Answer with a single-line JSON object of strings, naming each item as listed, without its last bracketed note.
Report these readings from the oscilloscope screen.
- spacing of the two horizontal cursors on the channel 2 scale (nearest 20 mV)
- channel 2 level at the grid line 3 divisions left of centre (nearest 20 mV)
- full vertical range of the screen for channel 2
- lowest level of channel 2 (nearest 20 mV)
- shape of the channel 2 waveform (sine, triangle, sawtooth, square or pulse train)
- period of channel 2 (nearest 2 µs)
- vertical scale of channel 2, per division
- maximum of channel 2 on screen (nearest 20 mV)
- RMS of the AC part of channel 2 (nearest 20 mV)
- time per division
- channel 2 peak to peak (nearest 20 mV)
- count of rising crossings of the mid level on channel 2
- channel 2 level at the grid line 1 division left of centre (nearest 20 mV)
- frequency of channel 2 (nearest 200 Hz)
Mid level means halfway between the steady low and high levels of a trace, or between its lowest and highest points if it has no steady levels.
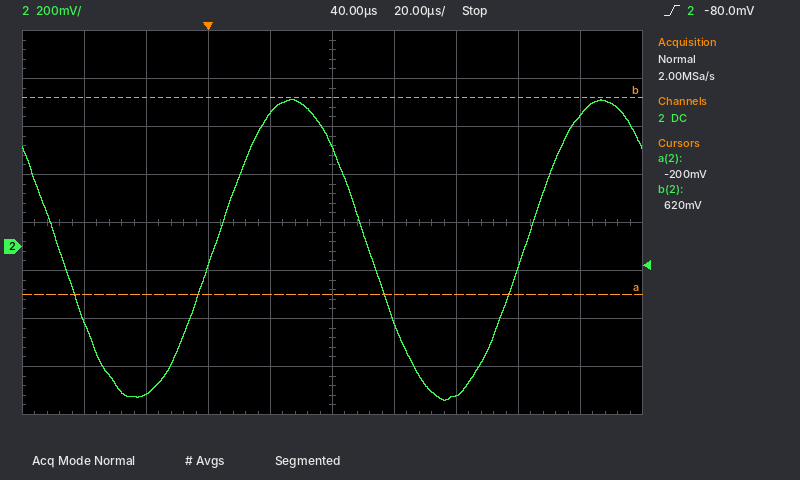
{"spacing of the two horizontal cursors on the channel 2 scale": "820 mV", "channel 2 level at the grid line 3 divisions left of centre": "-620 mV", "full vertical range of the screen for channel 2": "1.6 V", "lowest level of channel 2": "-640 mV", "shape of the channel 2 waveform": "sine", "period of channel 2": "100 µs", "vertical scale of channel 2, per division": "200 mV", "maximum of channel 2 on screen": "620 mV", "RMS of the AC part of channel 2": "440 mV", "time per division": "20 µs", "channel 2 peak to peak": "1.26 V", "count of rising crossings of the mid level on channel 2": "2", "channel 2 level at the grid line 1 division left of centre": "560 mV", "frequency of channel 2": "10.0 kHz"}
